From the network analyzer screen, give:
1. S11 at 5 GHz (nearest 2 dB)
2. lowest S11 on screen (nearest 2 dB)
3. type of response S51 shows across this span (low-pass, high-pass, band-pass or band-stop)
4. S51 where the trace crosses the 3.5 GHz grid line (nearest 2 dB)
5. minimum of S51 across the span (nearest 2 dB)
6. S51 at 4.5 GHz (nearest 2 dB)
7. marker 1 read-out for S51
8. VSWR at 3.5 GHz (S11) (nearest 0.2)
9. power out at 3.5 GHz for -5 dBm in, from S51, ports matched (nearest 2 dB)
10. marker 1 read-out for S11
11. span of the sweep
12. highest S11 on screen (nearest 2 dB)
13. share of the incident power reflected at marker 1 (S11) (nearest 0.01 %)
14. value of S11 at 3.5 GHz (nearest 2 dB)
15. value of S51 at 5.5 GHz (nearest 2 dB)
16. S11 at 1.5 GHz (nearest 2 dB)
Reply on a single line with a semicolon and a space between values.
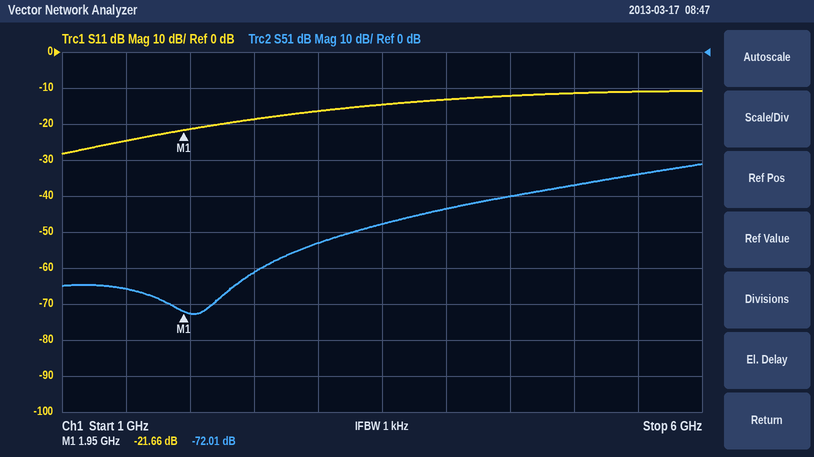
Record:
-12 dB; -28 dB; high-pass; -48 dB; -72 dB; -40 dB; -72.01 dB; 1.4; -52 dBm; -21.66 dB; 5 GHz; -10 dB; 0.68 %; -14 dB; -34 dB; -24 dB
